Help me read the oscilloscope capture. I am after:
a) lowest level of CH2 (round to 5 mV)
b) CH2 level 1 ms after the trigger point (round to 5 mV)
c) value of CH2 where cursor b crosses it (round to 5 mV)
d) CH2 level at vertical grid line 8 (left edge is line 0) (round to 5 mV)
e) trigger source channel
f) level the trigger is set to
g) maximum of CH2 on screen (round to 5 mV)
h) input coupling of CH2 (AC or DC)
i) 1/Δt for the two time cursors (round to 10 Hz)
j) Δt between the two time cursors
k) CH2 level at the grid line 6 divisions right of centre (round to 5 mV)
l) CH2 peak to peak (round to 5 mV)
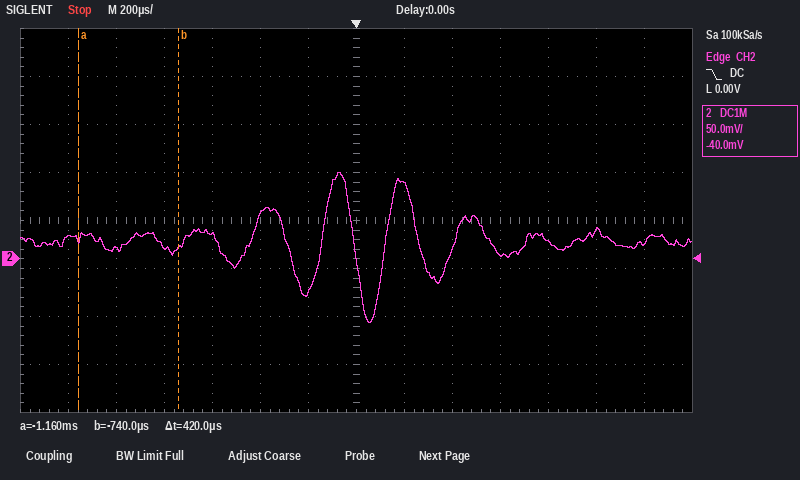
-65 mV
30 mV
10 mV
80 mV
CH2
0.00 V
90 mV
DC
2.38 kHz
420 µs
15 mV
155 mV
